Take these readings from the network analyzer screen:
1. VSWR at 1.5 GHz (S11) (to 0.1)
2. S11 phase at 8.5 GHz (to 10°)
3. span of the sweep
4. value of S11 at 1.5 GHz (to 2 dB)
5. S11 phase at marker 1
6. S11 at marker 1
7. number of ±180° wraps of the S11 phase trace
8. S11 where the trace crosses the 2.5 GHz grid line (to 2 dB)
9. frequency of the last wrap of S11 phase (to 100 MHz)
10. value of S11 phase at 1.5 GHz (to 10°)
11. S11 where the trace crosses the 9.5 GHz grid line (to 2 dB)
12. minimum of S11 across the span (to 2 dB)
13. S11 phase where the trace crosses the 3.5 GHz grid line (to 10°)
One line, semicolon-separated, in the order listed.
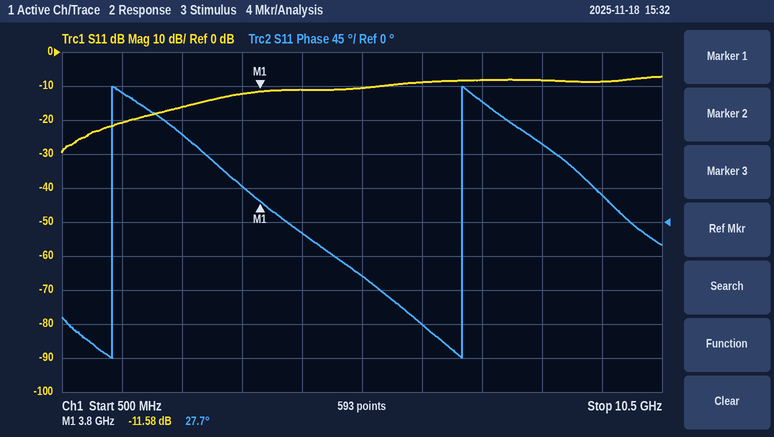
1.2; 100°; 10 GHz; -20 dB; 27.7°; -11.58 dB; 2; -16 dB; 7.2 GHz; 170°; -8 dB; -30 dB; 50°
